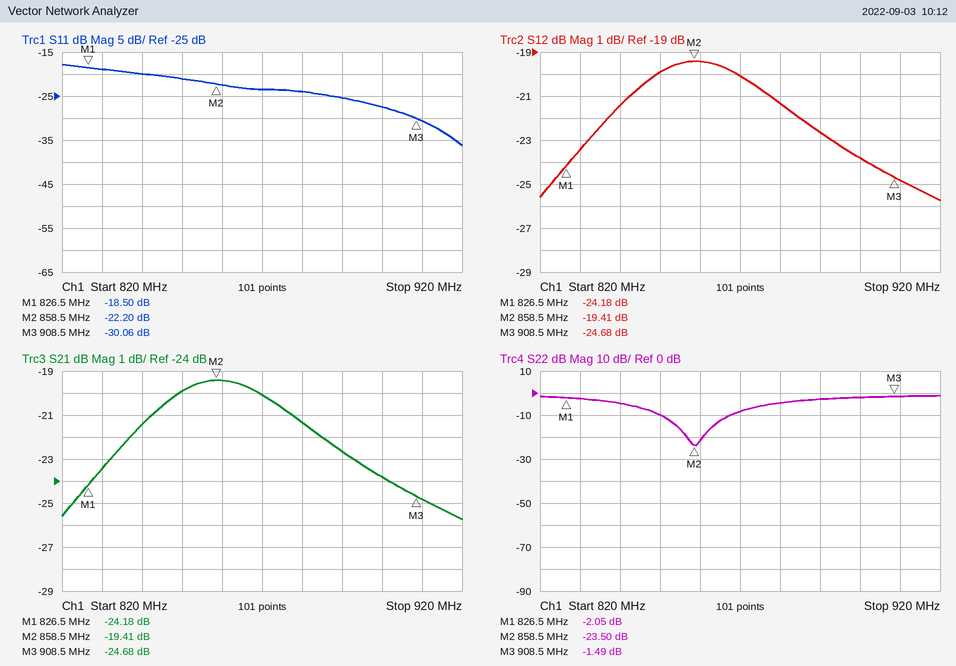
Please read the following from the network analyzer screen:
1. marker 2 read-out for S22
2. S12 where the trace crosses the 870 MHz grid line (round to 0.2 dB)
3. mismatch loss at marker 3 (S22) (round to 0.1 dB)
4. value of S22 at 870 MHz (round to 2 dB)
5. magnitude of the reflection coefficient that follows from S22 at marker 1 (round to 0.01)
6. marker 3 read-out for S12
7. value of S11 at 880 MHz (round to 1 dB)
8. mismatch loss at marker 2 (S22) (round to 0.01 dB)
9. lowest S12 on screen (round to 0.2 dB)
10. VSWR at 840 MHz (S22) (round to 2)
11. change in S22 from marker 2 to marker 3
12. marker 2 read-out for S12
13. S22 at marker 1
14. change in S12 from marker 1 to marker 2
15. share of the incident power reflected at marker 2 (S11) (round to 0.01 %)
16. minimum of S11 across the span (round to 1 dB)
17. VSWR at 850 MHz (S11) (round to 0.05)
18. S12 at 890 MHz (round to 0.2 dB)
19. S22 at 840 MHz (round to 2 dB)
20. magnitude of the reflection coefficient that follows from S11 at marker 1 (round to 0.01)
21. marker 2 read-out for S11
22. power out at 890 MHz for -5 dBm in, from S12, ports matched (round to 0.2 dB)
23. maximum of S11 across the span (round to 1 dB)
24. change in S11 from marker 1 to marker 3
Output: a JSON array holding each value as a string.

["-23.50 dB", "-20.0 dB", "5.4 dB", "-8 dB", "0.79", "-24.68 dB", "-24 dB", "0.02 dB", "-25.8 dB", "4", "22.01 dB", "-19.41 dB", "-2.05 dB", "4.77 dB", "0.60 %", "-36 dB", "1.20", "-22.6 dB", "-4 dB", "0.12", "-22.20 dB", "-27.6 dBm", "-18 dB", "-11.56 dB"]
